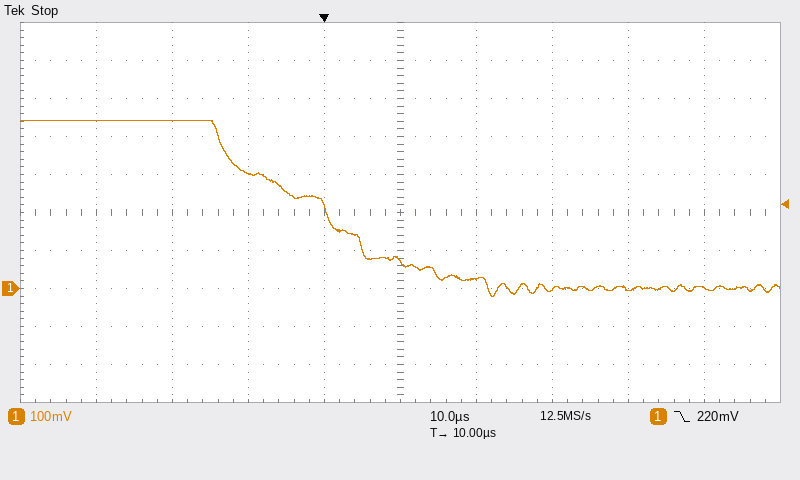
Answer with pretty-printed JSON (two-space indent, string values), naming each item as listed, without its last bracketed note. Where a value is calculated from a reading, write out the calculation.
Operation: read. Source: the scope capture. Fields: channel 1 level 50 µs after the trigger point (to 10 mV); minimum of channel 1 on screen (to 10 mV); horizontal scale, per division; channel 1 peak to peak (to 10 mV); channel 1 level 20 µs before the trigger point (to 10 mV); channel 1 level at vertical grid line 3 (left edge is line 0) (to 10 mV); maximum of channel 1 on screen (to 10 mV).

{
  "channel 1 level 50 µs after the trigger point": "0 mV",
  "minimum of channel 1 on screen": "-20 mV",
  "horizontal scale, per division": "10 µs",
  "channel 1 peak to peak": "440 mV − (-20 mV) = 460 mV",
  "channel 1 level 20 µs before the trigger point": "440 mV",
  "channel 1 level at vertical grid line 3 (left edge is line 0)": "300 mV",
  "maximum of channel 1 on screen": "440 mV"
}
